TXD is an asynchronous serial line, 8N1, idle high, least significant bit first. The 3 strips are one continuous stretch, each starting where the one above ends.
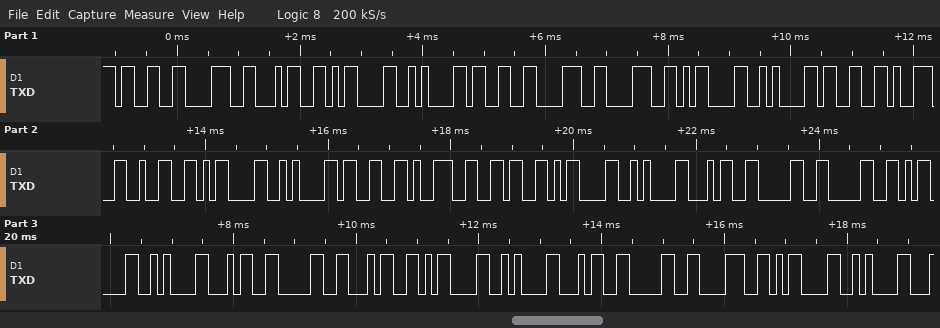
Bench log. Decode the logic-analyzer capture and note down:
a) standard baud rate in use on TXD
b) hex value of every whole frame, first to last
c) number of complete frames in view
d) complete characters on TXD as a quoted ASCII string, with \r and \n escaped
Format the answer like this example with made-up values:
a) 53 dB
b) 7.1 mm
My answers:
a) 9600 baud
b) 33 38 34 0D 0A 33 38 38 0D 0A 33 39 32 0D 0A 33 39 36 0D 0A 34 30 30 0D 0A 34 30 34 0D 0A 34 30 38 0D 0A
c) 35
d) "384\r\n388\r\n392\r\n396\r\n400\r\n404\r\n408\r\n"
